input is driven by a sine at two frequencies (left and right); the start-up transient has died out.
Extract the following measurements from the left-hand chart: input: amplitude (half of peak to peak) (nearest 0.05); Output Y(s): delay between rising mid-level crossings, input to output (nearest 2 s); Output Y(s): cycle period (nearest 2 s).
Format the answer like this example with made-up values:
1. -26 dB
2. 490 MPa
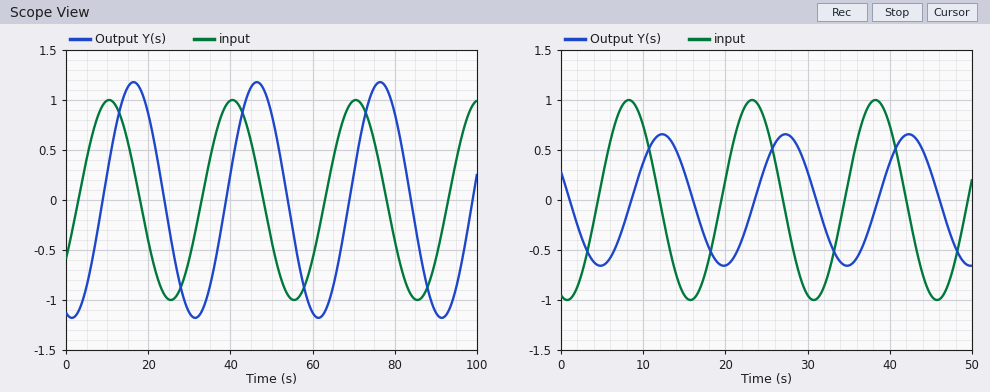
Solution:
1. 1.00
2. 6 s
3. 30 s
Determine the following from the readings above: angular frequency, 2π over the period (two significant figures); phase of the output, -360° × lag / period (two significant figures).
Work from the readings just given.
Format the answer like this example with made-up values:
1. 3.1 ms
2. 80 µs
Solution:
1. 0.21 rad/s
2. -72°
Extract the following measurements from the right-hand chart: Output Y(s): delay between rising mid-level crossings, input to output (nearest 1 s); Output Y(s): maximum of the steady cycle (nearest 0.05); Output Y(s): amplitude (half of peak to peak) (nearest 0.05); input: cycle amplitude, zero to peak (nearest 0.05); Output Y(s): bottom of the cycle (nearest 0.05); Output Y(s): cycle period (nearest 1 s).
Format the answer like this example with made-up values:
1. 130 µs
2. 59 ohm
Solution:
1. 4 s
2. 0.65
3. 0.65
4. 1.00
5. -0.65
6. 15 s
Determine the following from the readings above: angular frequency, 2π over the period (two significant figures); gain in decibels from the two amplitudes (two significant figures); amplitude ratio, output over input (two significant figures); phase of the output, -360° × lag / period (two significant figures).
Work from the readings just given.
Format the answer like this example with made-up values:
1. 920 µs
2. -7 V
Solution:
1. 0.42 rad/s
2. -3.7 dB
3. 0.65
4. -96°
